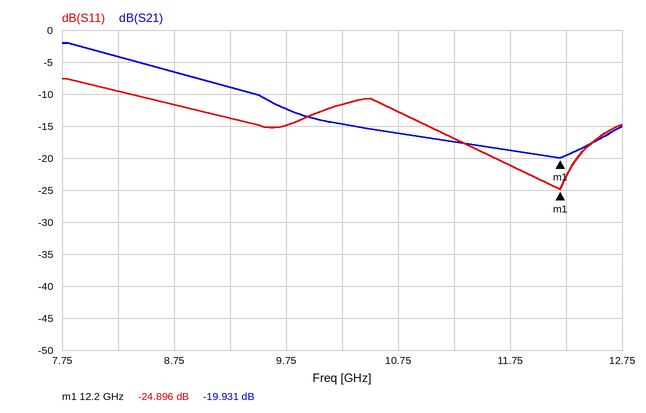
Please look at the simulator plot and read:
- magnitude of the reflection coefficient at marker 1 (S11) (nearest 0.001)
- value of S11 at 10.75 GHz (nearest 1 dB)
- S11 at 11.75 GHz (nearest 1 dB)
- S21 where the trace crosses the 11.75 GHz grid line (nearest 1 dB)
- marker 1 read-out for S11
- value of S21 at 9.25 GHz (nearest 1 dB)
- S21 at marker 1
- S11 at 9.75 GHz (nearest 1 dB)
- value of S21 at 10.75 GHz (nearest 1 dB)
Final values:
0.057
-13 dB
-21 dB
-19 dB
-24.896 dB
-9 dB
-19.931 dB
-15 dB
-16 dB
